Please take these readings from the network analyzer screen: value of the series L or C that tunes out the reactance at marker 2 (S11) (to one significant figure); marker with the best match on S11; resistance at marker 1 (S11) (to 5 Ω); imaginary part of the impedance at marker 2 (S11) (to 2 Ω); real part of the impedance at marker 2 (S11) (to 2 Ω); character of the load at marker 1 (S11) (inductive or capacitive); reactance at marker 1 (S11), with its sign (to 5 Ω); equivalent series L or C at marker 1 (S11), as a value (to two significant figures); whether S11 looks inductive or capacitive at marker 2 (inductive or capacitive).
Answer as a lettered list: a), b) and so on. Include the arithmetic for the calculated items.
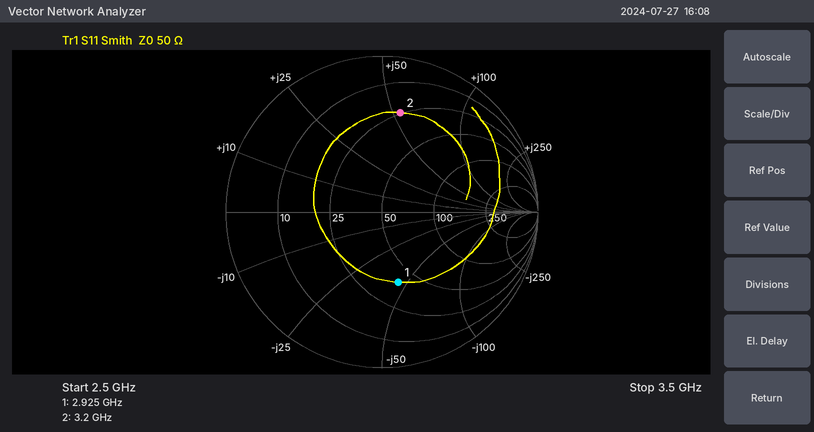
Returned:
a) C = 1/(2π × 3.2 GHz × 54 Ω) ≈ 921 fF, so 900 fF to one significant figure
b) marker 1
c) 40 Ω
d) +54 Ω
e) 24 Ω
f) capacitive
g) -45 Ω
h) C = 1/(2π × 2.925 GHz × 45 Ω) ≈ 1.2 pF
i) inductive
